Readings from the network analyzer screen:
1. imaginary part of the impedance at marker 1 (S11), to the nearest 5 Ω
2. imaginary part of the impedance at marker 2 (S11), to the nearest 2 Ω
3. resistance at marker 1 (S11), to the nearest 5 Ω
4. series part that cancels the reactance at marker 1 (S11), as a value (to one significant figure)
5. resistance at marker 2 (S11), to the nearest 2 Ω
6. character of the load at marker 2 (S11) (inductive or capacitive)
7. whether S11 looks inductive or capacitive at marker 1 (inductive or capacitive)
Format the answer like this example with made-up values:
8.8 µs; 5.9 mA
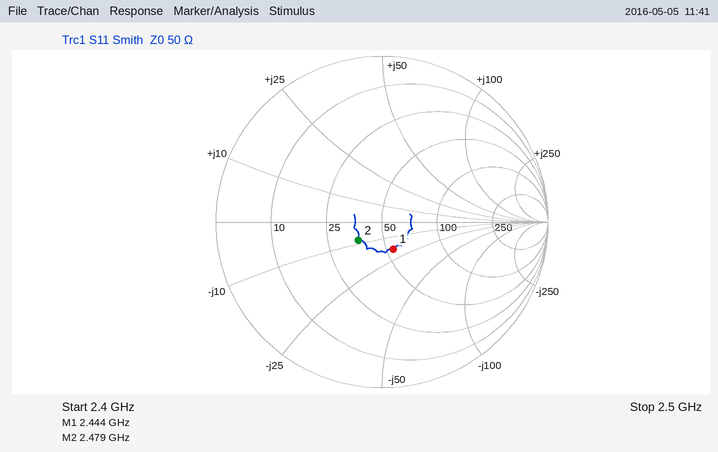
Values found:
-20 Ω; -8 Ω; 55 Ω; 1 nH; 36 Ω; capacitive; capacitive
